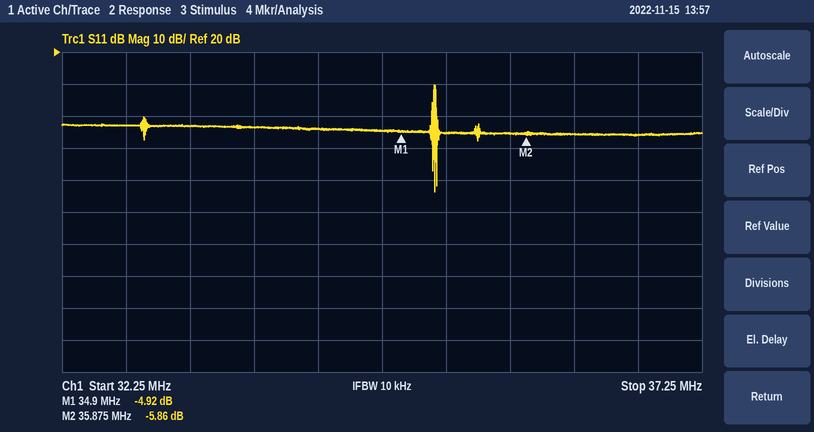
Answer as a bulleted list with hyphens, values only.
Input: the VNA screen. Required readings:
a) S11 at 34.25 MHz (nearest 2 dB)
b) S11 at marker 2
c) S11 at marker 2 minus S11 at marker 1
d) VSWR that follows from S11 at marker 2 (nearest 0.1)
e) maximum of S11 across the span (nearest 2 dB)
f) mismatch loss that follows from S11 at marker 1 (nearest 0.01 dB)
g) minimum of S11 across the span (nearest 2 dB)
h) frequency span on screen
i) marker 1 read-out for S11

- -4 dB
- -5.86 dB
- -0.94 dB
- 3.1
- 10 dB
- 1.69 dB
- -24 dB
- 5 MHz
- -4.92 dB
